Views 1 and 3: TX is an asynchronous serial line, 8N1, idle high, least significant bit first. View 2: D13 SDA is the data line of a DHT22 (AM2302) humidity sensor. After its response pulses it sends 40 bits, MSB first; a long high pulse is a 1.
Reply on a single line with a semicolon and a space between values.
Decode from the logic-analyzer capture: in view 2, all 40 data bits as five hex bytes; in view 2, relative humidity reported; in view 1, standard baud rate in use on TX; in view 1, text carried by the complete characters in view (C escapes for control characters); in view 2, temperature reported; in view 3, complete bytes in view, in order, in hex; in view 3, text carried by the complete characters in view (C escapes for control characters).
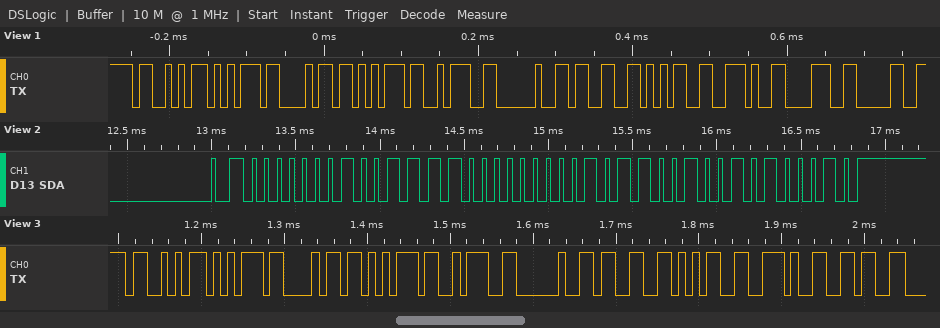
01 3C 01 64 A2; 31.6 %; 115200 baud; "Suhu: 35.80"; 35.6 °C; 53 75 68 75 3A 20 33 35 2E 36; "Suhu: 35.6"
